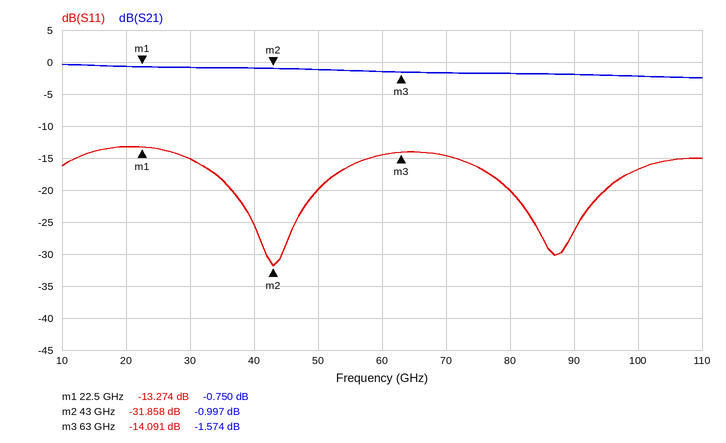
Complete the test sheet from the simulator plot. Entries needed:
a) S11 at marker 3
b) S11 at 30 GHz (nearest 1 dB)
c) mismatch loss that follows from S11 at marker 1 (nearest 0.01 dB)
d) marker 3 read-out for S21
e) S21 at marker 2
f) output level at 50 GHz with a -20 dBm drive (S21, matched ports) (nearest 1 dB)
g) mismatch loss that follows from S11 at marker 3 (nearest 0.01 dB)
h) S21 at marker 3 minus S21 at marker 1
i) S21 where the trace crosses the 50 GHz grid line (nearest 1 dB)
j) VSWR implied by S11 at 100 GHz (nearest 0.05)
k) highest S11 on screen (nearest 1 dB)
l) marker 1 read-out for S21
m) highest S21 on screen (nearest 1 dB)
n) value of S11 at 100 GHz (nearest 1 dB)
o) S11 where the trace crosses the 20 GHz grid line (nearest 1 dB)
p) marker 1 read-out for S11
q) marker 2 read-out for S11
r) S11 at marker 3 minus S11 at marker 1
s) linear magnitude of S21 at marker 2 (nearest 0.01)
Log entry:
-14.091 dB
-15 dB
0.21 dB
-1.574 dB
-0.997 dB
-21 dBm
0.17 dB
-0.824 dB
-1 dB
1.35
-13 dB
-0.750 dB
0 dB
-17 dB
-13 dB
-13.274 dB
-31.858 dB
-0.817 dB
0.89
